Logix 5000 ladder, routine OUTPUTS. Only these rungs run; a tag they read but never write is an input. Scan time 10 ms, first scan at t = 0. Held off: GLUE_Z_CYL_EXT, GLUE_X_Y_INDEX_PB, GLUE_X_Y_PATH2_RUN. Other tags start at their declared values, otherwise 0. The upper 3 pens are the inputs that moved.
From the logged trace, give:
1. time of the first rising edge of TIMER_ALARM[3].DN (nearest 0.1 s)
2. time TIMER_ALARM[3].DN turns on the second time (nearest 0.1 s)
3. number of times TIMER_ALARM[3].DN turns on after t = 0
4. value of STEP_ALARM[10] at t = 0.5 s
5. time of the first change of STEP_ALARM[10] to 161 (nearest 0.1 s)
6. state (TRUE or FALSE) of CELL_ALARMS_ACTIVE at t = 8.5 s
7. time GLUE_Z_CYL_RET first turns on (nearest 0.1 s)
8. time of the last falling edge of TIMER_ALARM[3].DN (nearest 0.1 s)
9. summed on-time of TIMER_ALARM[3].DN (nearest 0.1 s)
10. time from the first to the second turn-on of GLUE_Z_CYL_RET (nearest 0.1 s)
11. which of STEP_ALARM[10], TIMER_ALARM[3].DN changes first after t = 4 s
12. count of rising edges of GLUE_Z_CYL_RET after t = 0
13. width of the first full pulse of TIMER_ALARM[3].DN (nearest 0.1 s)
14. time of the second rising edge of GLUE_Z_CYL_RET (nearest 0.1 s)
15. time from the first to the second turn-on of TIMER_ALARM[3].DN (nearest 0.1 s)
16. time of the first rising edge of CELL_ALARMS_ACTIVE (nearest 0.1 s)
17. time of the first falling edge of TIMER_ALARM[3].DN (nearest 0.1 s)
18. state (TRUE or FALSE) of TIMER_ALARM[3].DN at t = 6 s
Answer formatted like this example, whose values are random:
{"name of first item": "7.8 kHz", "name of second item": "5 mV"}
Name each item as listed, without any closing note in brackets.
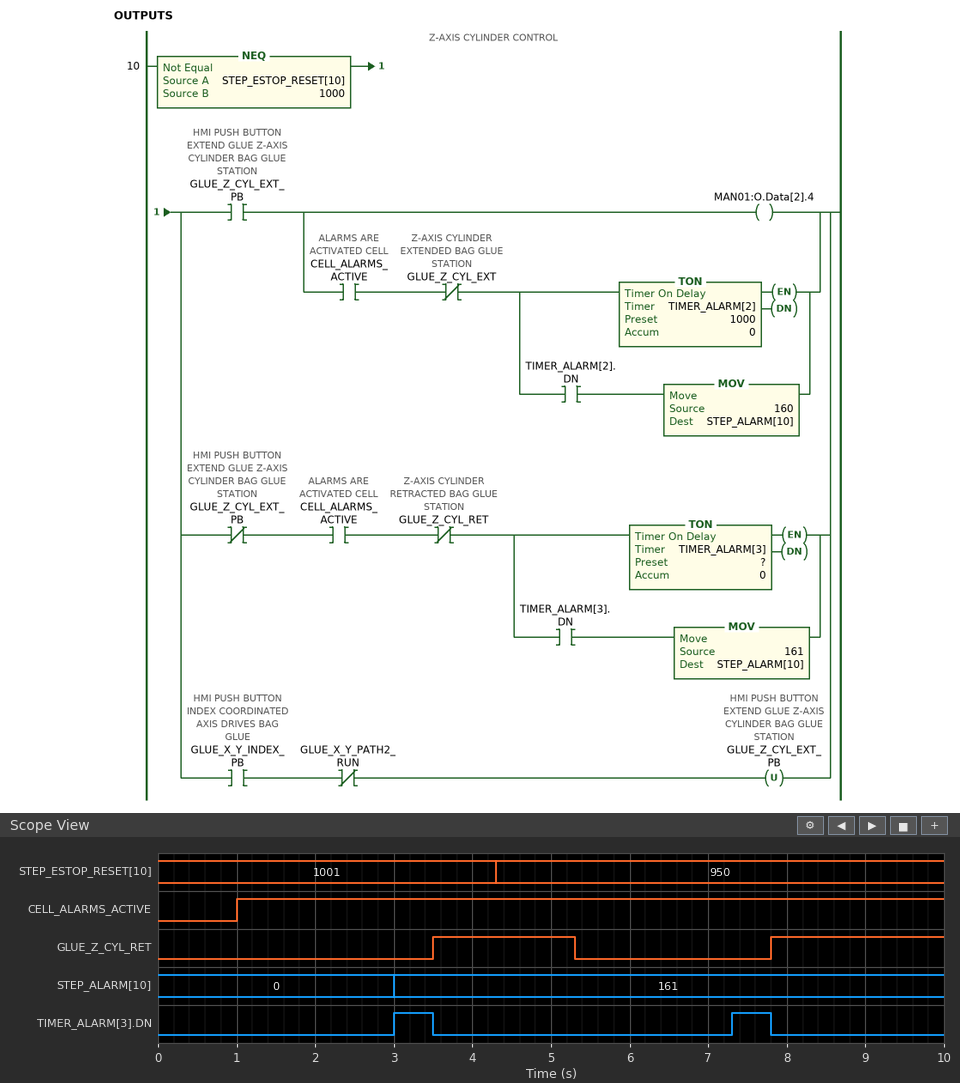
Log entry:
{"time of the first rising edge of TIMER_ALARM[3].DN": "3.0 s", "time TIMER_ALARM[3].DN turns on the second time": "7.3 s", "number of times TIMER_ALARM[3].DN turns on after t = 0": "2", "value of STEP_ALARM[10] at t = 0.5 s": "0", "time of the first change of STEP_ALARM[10] to 161": "3.0 s", "state (TRUE or FALSE) of CELL_ALARMS_ACTIVE at t = 8.5 s": "TRUE", "time GLUE_Z_CYL_RET first turns on": "3.5 s", "time of the last falling edge of TIMER_ALARM[3].DN": "7.8 s", "summed on-time of TIMER_ALARM[3].DN": "1.0 s", "time from the first to the second turn-on of GLUE_Z_CYL_RET": "4.3 s", "which of STEP_ALARM[10], TIMER_ALARM[3].DN changes first after t = 4 s": "TIMER_ALARM[3].DN", "count of rising edges of GLUE_Z_CYL_RET after t = 0": "2", "width of the first full pulse of TIMER_ALARM[3].DN": "0.5 s", "time of the second rising edge of GLUE_Z_CYL_RET": "7.8 s", "time from the first to the second turn-on of TIMER_ALARM[3].DN": "4.3 s", "time of the first rising edge of CELL_ALARMS_ACTIVE": "1.0 s", "time of the first falling edge of TIMER_ALARM[3].DN": "3.5 s", "state (TRUE or FALSE) of TIMER_ALARM[3].DN at t = 6 s": "FALSE"}
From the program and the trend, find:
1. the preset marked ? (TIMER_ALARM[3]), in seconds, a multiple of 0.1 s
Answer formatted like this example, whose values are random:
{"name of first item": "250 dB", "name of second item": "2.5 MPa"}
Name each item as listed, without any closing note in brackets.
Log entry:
{"the preset marked ? (TIMER_ALARM[3]), in seconds, a multiple of 0.1 s": "2.0 s"}
